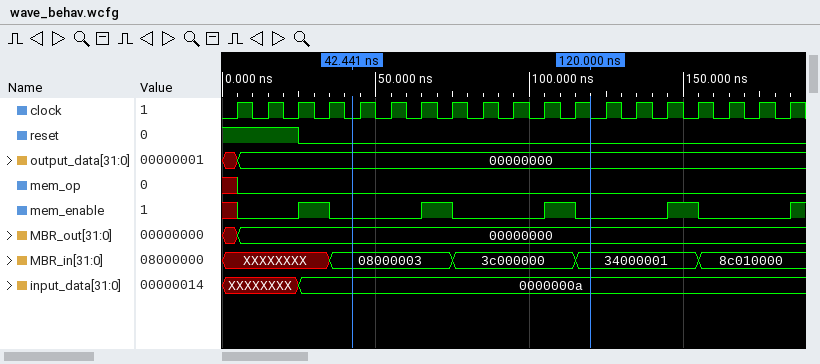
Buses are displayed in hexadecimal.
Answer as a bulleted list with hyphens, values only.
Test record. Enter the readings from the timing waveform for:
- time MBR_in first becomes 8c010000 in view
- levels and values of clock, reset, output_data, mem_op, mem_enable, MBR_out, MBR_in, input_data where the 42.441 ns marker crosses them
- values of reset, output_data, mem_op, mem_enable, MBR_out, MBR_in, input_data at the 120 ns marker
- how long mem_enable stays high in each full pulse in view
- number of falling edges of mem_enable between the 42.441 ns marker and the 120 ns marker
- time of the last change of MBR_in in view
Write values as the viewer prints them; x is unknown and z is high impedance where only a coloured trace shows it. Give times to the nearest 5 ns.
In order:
- 155 ns
- clock=0, reset=0, output_data=00000000, mem_op=0, mem_enable=0, MBR_out=00000000, MBR_in=08000003, input_data=0000000a
- reset=0, output_data=00000000, mem_op=0, mem_enable=0, MBR_out=00000000, MBR_in=34000001, input_data=0000000a
- 10 ns, 10 ns, 10 ns, 10 ns
- 2
- 155 ns
